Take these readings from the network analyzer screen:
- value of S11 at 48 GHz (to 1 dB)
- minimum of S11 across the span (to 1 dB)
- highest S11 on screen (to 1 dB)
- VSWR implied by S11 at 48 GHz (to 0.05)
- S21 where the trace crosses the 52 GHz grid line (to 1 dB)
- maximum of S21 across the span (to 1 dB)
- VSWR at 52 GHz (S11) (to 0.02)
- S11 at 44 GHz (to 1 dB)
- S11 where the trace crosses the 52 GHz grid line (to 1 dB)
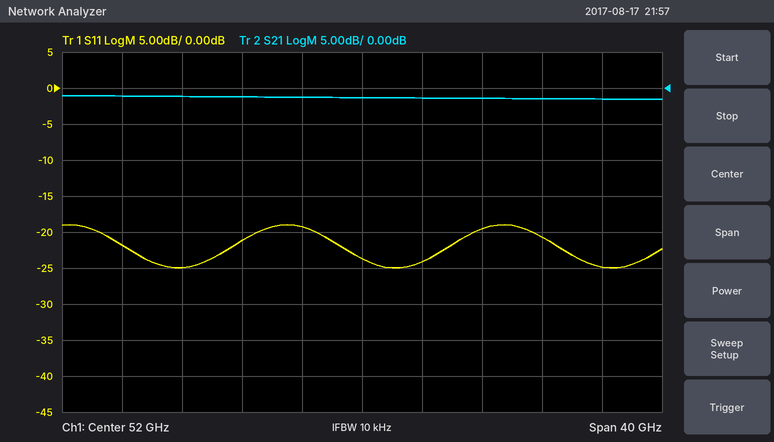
-19 dB
-25 dB
-19 dB
1.25
-1 dB
-1 dB
1.14
-21 dB
-24 dB
